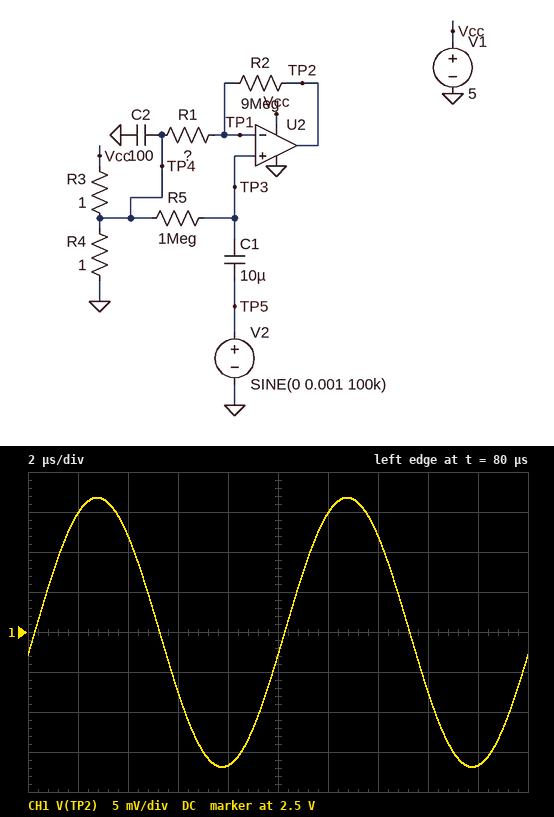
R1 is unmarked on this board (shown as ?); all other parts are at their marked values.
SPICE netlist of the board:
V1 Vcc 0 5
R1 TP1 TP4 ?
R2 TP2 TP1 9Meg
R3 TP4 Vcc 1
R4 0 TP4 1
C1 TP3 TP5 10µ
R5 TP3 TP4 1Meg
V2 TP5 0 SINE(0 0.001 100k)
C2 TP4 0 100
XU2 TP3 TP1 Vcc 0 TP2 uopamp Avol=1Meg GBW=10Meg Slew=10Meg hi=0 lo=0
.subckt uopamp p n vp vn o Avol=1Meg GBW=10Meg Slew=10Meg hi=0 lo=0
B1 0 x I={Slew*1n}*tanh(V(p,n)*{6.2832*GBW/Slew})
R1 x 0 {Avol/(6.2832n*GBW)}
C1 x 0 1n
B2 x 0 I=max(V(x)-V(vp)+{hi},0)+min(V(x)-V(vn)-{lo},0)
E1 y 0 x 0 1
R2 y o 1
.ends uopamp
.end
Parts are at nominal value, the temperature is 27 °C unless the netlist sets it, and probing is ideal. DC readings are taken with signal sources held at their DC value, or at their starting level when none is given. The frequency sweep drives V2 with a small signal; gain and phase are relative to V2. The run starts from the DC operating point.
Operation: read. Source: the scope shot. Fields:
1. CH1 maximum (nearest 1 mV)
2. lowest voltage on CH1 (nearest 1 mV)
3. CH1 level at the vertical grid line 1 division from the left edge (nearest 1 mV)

2.517 V
2.483 V
2.515 V
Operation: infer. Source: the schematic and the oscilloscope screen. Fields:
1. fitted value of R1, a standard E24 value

560 kΩ
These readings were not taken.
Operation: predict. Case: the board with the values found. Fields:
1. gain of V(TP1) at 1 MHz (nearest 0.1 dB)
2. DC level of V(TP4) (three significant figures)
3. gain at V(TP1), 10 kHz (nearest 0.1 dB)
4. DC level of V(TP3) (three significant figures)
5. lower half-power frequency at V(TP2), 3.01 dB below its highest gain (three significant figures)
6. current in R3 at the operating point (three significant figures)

-5.9 dB
2.50 V
0 dB
2.50 V
15.9 mHz
2.50 A
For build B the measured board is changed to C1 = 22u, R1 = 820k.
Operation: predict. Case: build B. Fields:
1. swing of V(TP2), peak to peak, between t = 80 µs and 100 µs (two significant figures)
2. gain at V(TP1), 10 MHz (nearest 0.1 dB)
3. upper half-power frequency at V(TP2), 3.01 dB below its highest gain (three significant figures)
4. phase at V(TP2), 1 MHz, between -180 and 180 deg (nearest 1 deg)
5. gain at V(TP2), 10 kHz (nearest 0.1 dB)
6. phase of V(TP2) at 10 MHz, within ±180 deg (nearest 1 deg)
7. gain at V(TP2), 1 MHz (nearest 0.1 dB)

24 mV
-21.6 dB
835 kHz
-50 deg
21.6 dB
-85 deg
17.7 dB
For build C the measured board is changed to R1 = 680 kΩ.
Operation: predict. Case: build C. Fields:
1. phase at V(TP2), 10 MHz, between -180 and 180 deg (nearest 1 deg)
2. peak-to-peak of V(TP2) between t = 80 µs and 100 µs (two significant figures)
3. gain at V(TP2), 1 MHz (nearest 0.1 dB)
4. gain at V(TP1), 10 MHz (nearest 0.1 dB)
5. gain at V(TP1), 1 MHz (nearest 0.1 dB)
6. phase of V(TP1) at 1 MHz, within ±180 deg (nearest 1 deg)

-86 deg
28 mV
18.3 dB
-23.1 dB
-4.8 dB
-55 deg
